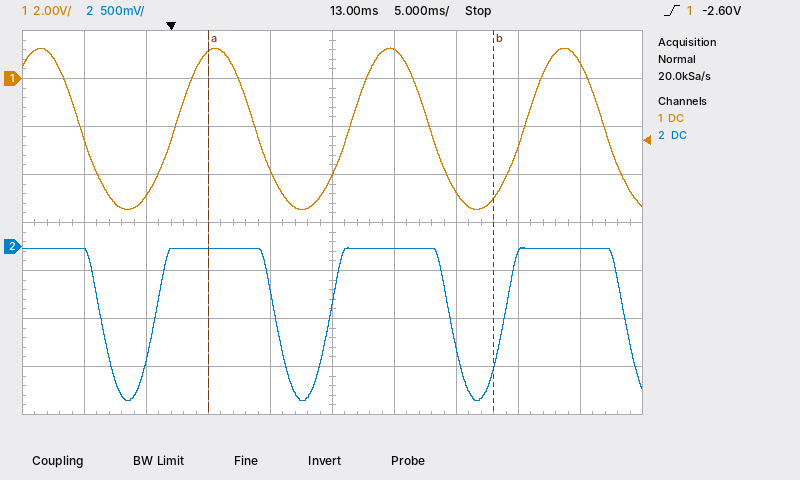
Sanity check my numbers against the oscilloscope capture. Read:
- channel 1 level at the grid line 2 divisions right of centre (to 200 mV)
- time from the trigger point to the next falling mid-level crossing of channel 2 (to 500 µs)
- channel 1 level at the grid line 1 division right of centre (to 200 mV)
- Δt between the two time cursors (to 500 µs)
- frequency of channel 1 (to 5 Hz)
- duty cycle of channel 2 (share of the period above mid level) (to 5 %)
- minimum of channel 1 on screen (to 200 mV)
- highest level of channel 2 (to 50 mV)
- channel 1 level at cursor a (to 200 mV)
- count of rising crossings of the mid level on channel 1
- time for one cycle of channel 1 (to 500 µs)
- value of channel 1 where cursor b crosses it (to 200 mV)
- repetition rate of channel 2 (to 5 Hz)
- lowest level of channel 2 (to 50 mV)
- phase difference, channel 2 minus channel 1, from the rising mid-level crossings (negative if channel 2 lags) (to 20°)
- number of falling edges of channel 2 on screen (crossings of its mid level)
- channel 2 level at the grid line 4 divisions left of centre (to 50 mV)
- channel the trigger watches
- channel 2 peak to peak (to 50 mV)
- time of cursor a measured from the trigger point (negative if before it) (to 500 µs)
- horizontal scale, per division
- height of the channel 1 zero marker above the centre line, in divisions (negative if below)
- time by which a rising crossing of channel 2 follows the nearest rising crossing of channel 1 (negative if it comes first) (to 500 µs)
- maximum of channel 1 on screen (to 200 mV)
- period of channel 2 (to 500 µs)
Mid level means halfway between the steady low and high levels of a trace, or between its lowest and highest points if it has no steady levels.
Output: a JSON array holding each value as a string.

["-4.8 V", "8.5 ms", "1.2 V", "23.0 ms", "70 Hz", "70 %", "-5.4 V", "0 mV", "1.2 V", "3", "14.0 ms", "-5.0 V", "70 Hz", "-1.60 V", "+40°", "4", "-50 mV", "channel 1", "1.60 V", "+3.0 ms", "5 ms", "+3.0 div", "-1.5 ms", "1.2 V", "14.0 ms"]
